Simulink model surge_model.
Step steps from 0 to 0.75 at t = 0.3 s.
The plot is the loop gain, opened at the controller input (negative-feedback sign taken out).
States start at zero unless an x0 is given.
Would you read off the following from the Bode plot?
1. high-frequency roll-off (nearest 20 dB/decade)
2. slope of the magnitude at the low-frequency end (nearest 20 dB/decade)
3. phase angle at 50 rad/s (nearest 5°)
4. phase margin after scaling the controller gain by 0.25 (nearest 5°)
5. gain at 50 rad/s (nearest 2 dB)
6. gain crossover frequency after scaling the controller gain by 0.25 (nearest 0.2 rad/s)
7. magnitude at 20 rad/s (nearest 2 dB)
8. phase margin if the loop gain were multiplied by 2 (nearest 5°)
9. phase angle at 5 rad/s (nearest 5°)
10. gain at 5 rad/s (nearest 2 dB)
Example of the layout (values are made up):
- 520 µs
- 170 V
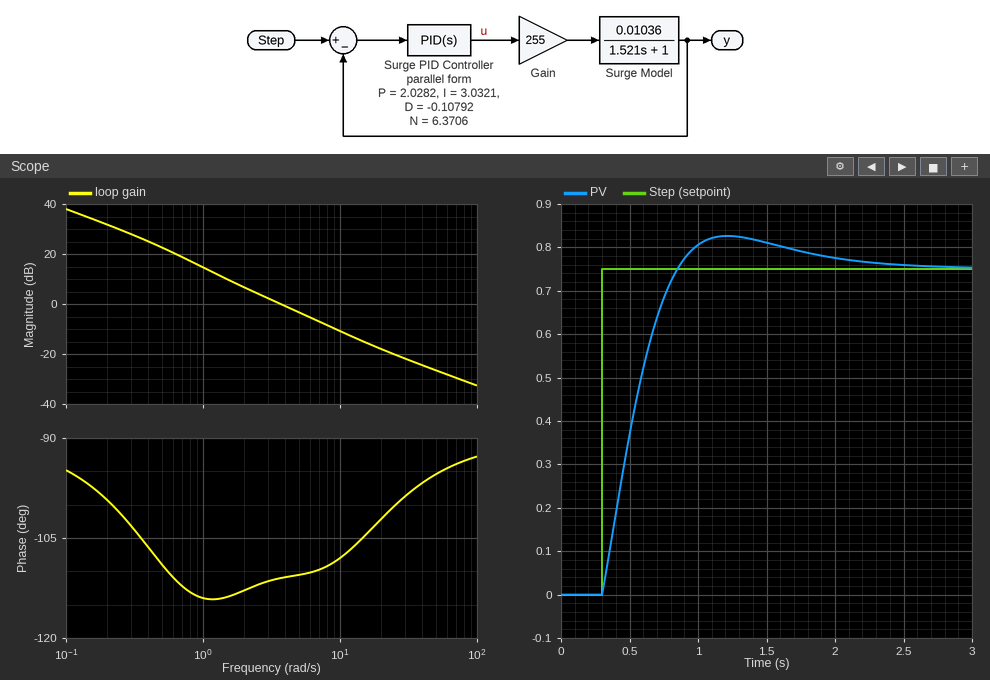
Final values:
- -20 dB/decade
- -20 dB/decade
- -95°
- 65°
- -26 dB
- 1.2 rad/s
- -18 dB
- 70°
- -110°
- -4 dB
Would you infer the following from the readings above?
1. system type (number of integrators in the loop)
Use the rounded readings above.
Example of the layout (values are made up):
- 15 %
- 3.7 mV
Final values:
- 1
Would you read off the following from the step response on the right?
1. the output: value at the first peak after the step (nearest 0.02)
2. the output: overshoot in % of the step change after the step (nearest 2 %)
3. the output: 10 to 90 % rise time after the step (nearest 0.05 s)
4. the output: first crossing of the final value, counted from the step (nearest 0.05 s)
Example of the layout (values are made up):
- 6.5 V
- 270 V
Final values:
- 0.82
- 10 %
- 0.40 s
- 0.55 s
